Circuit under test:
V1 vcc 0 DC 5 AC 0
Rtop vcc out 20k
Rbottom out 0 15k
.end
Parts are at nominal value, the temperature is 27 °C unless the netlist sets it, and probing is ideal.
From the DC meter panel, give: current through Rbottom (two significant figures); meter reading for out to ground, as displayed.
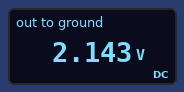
140 µA
2.143 V
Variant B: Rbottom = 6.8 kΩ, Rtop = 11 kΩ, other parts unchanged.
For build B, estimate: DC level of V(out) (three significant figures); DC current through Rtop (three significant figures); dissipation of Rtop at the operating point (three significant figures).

1.91 V
281 µA
868 µW
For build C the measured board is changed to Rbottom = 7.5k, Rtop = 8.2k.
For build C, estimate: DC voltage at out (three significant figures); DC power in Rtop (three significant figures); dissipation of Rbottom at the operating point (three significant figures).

2.39 V
832 µW
761 µW
